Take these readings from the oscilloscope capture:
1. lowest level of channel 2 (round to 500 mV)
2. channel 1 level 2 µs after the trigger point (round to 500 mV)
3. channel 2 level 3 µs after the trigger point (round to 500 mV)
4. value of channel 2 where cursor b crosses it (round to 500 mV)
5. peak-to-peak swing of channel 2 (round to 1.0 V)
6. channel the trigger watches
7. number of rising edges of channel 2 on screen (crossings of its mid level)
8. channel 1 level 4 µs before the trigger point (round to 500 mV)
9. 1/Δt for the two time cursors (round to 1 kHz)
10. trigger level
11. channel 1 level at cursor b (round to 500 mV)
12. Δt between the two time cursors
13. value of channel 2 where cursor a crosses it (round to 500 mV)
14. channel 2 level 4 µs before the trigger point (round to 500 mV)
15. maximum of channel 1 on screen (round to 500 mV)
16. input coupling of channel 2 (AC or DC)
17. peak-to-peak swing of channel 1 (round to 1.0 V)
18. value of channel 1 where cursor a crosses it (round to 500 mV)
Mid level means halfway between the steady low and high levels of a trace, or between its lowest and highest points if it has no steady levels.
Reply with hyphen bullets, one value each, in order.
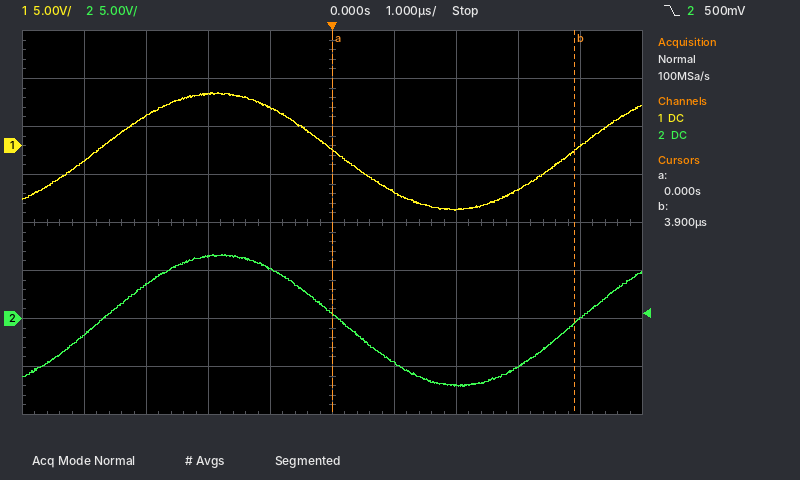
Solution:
- -7.0 V
- -6.5 V
- -5.0 V
- -500 mV
- 14.0 V
- channel 2
- 2
- -1.5 V
- 256 kHz
- 500 mV
- -500 mV
- 3.9 µs
- 500 mV
- -1.5 V
- 5.5 V
- DC
- 12.0 V
- -500 mV
